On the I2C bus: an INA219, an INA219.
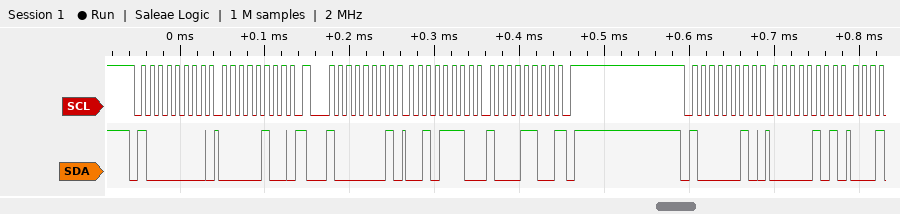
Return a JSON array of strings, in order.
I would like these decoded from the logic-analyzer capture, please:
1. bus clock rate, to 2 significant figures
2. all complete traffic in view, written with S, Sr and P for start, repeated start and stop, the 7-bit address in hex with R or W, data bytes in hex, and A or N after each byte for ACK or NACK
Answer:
["100 kHz", "S 40W A 04 A Sr 40R A 2E A 8C N P S 41W A 05 A"]
